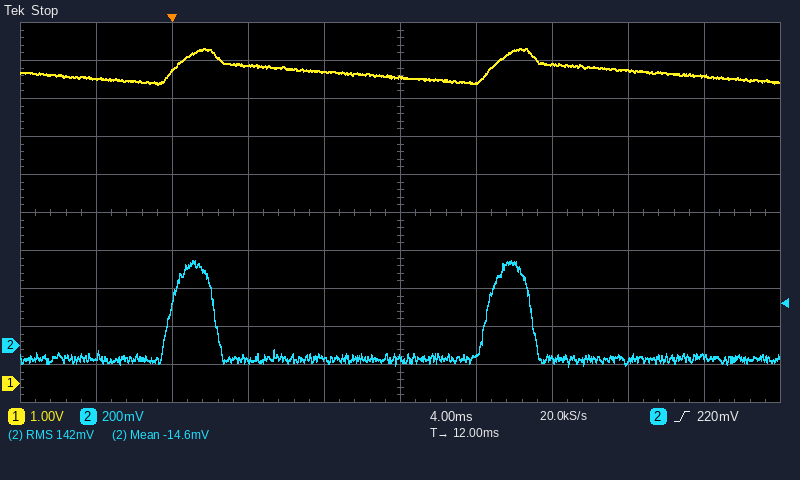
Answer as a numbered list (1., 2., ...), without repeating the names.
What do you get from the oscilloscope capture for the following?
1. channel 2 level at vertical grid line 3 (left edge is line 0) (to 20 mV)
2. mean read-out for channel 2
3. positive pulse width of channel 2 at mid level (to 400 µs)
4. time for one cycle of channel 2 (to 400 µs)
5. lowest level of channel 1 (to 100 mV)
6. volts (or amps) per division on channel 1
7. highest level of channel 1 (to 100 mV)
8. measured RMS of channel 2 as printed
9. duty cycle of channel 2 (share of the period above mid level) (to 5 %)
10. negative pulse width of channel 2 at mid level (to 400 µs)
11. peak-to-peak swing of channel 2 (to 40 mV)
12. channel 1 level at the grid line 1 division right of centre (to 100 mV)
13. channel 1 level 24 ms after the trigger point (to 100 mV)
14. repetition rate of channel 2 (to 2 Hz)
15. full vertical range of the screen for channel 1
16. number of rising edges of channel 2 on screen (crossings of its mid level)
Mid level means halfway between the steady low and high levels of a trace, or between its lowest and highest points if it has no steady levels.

1. -80 mV
2. -14.6 mV
3. 2.4 ms
4. 16.8 ms
5. 7.9 V
6. 1 V
7. 8.8 V
8. 142 mV
9. 15 %
10. 14.4 ms
11. 560 mV
12. 7.9 V
13. 8.2 V
14. 60 Hz
15. 10 V
16. 2
